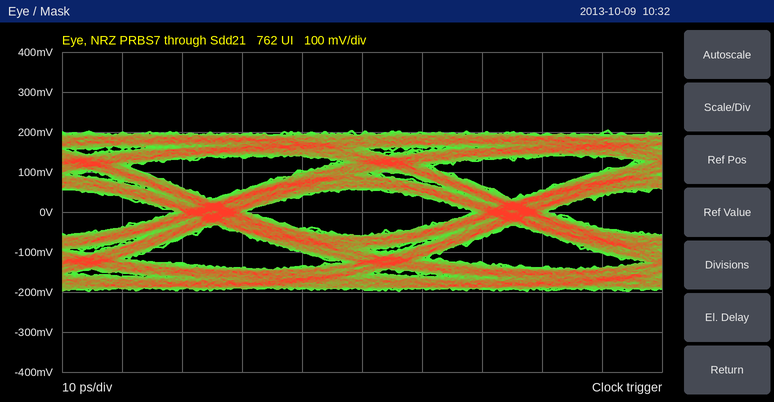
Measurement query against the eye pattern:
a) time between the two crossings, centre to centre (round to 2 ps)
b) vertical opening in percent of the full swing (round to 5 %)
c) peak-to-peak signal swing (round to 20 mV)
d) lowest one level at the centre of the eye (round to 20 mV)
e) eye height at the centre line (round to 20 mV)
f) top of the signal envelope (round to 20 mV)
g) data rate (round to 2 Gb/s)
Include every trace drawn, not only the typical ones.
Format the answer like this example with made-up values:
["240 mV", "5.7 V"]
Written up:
["50 ps", "30 %", "400 mV", "60 mV", "120 mV", "200 mV", "20 Gb/s"]
